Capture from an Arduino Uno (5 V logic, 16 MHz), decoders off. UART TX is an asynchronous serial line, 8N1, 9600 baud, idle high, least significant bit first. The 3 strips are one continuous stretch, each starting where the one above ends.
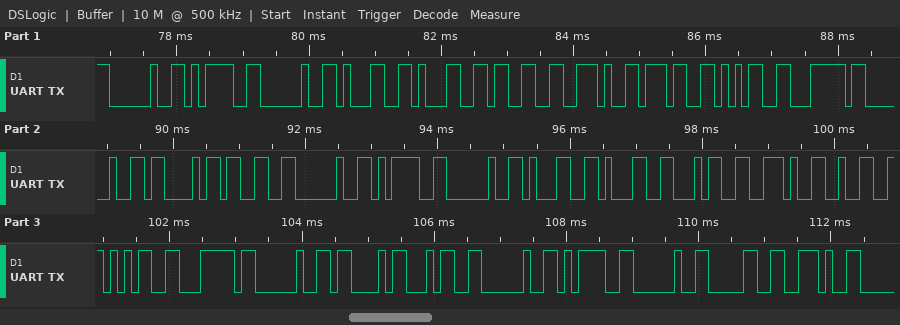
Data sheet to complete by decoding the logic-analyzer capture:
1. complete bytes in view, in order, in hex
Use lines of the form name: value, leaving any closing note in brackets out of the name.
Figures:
complete bytes in view, in order, in hex: 20 3D 20 31 31 33 2E 37 35 7C 20 43 33 20 3D 20 31 31 34 2E 32 35 7C 20 43 34 20 3D 20 30 2E
